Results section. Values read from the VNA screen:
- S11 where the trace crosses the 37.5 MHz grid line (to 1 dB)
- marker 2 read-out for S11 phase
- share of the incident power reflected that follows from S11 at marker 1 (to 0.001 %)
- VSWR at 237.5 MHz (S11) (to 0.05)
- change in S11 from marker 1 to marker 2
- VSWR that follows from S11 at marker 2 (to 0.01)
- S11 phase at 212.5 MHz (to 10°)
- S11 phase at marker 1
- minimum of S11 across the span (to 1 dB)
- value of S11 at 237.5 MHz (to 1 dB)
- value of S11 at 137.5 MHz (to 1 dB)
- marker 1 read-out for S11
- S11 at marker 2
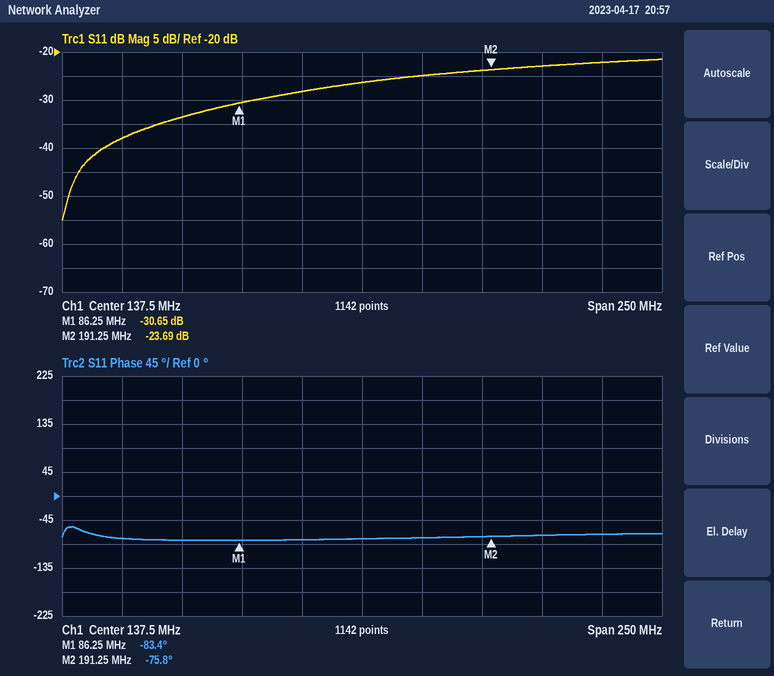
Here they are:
-38 dB
-75.8°
0.086 %
1.15
6.96 dB
1.14
-70°
-83.4°
-55 dB
-22 dB
-26 dB
-30.65 dB
-23.69 dB
